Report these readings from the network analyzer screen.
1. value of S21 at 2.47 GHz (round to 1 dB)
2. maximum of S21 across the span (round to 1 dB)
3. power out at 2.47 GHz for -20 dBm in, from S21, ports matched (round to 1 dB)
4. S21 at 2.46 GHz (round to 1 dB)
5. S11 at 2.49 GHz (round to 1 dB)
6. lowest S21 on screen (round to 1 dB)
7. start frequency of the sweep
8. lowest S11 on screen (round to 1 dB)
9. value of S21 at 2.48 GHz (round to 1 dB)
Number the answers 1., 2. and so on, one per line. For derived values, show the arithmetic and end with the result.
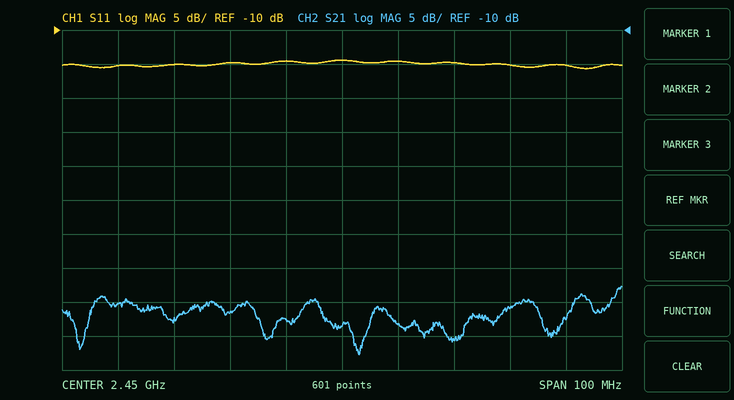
1. -56 dB
2. -48 dB
3. -20 dBm + (-56 dB) = -76 dBm
4. -53 dB
5. -15 dB
6. -58 dB
7. 2.4 GHz
8. -16 dB
9. -51 dB
